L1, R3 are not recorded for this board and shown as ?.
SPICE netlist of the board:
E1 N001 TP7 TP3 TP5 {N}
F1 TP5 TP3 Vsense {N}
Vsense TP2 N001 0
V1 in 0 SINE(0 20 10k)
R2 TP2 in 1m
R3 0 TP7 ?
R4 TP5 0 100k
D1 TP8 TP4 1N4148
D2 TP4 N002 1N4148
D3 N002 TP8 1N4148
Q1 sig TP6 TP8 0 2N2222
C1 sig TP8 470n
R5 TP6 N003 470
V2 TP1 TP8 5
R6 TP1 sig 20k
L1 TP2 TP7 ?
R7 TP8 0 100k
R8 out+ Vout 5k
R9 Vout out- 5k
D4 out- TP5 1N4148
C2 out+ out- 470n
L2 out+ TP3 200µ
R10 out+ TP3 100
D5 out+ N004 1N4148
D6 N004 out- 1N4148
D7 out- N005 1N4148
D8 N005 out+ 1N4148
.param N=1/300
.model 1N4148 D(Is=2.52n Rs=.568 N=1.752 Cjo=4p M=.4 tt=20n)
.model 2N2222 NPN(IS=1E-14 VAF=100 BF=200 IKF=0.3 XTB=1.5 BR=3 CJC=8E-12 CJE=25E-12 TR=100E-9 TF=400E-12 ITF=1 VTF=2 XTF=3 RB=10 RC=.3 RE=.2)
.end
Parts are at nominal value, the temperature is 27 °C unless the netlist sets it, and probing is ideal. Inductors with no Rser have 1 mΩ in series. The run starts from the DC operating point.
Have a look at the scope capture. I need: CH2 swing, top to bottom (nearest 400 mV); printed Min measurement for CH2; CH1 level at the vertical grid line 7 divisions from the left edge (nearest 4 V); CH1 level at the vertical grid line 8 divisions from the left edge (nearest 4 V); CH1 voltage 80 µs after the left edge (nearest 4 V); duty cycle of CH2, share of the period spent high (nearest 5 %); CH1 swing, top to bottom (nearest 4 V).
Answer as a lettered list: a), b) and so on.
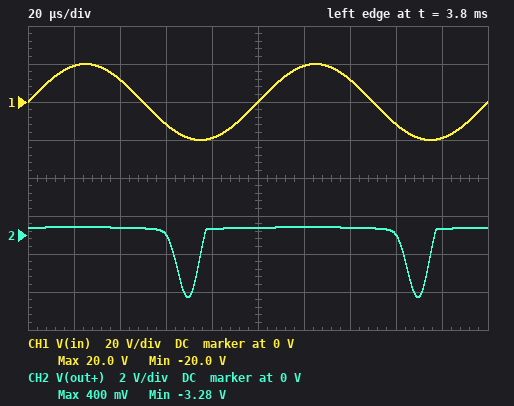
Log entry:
a) 3.6 V
b) -3.28 V
c) 12 V
d) -12 V
e) -20 V
f) 90 %
g) 40 V
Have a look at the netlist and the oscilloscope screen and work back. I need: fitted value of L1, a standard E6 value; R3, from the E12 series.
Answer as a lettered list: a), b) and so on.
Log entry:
a) 68 µH
b) 12 kΩ
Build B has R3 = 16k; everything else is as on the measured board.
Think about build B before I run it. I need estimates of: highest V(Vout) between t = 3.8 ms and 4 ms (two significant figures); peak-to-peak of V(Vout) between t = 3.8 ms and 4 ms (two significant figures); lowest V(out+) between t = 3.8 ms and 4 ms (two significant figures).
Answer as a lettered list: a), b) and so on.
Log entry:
a) 370 mV
b) 3.3 V
c) -2.9 V
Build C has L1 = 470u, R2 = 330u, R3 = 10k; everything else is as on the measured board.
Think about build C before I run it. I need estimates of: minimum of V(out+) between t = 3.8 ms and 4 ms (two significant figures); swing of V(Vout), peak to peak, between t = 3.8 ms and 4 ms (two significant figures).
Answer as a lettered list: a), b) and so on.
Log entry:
a) -2.7 V
b) 3.1 V
